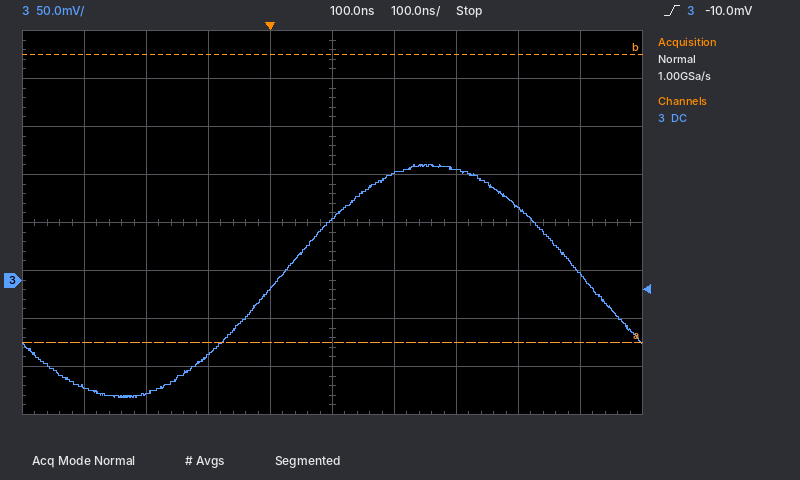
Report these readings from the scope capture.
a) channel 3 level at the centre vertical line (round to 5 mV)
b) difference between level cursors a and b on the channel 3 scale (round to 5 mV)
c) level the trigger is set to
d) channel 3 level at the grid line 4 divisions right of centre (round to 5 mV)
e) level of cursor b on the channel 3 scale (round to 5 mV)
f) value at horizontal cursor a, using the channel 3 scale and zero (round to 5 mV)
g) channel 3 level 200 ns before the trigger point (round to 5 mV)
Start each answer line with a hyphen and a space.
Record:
- 65 mV
- 300 mV
- -10.0 mV
- 5 mV
- 235 mV
- -65 mV
- -120 mV
